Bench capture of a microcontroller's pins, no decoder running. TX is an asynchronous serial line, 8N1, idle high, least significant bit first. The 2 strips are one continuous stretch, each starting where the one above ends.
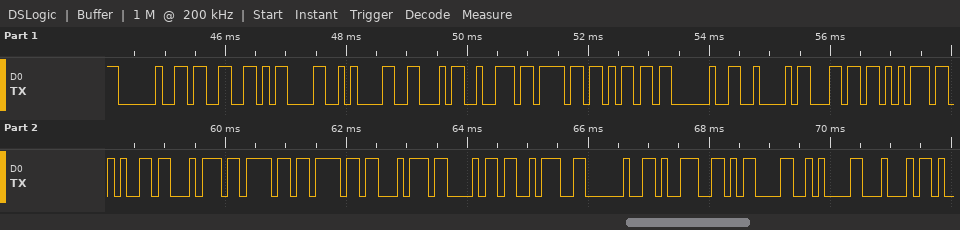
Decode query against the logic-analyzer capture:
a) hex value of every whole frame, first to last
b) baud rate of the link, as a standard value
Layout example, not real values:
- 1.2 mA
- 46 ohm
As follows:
- 20 33 0D 0A 46 72 6F 6D 20 42 6C 75 65 74 6F 6F 74 68 3A 20 39 0D 0A 44
- 9600 baud
